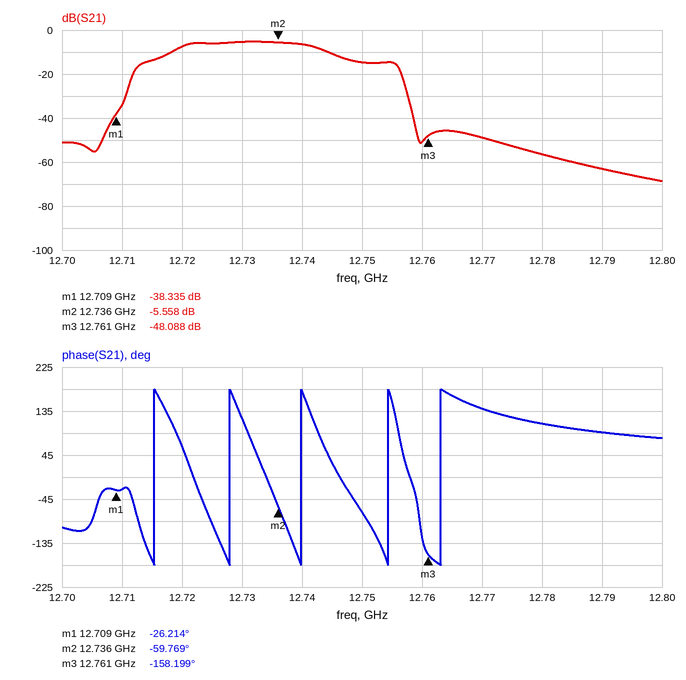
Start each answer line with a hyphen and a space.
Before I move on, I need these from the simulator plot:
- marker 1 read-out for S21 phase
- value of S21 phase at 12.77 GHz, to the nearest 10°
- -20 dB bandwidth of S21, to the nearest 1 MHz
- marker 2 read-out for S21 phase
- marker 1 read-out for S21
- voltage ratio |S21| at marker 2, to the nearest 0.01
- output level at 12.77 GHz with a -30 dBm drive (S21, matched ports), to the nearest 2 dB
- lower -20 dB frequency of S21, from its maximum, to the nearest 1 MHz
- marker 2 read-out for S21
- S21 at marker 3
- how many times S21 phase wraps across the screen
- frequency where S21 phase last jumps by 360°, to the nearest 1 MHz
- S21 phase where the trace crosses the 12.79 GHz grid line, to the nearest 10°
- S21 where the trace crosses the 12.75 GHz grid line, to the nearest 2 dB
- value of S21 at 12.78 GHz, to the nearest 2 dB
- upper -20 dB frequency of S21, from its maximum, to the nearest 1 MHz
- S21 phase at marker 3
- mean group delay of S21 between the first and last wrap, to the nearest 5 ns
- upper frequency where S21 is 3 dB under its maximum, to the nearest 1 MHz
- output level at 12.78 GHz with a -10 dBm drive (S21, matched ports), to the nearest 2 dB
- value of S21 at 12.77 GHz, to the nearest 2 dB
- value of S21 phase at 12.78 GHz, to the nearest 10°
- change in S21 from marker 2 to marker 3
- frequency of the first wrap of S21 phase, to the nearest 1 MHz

- -26.214°
- 140°
- 46 MHz
- -59.769°
- -38.335 dB
- 0.53
- -78 dBm
- 12.711 GHz
- -5.558 dB
- -48.088 dB
- 5
- 12.763 GHz
- 90°
- -14 dB
- -56 dB
- 12.757 GHz
- -158.199°
- 85 ns
- 12.743 GHz
- -66 dBm
- -48 dB
- 110°
- -42.530 dB
- 12.715 GHz
